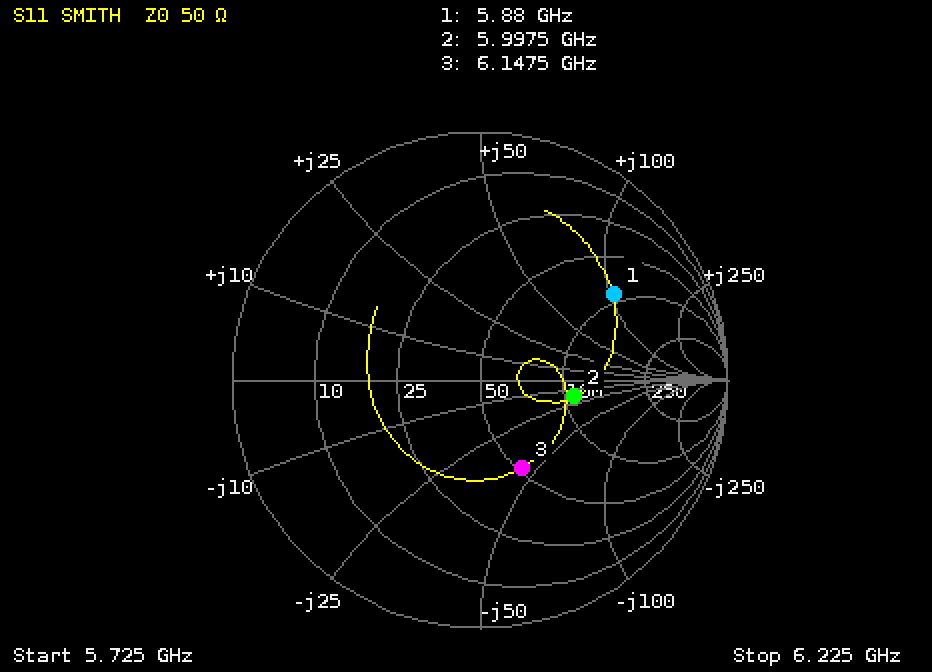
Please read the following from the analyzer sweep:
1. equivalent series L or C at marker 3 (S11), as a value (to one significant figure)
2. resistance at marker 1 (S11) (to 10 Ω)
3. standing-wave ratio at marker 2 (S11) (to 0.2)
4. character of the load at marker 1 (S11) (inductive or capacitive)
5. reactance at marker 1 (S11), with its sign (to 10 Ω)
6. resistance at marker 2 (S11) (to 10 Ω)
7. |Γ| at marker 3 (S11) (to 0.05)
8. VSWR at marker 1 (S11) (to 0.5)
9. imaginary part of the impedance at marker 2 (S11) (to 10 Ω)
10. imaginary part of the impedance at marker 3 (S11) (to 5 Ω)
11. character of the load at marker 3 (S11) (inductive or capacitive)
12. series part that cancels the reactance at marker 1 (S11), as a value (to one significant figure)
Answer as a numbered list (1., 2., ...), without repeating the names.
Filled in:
1. 600 fF
2. 90 Ω
3. 2.2
4. inductive
5. +100 Ω
6. 110 Ω
7. 0.40
8. 4.5
9. -20 Ω
10. -45 Ω
11. capacitive
12. 300 fF
